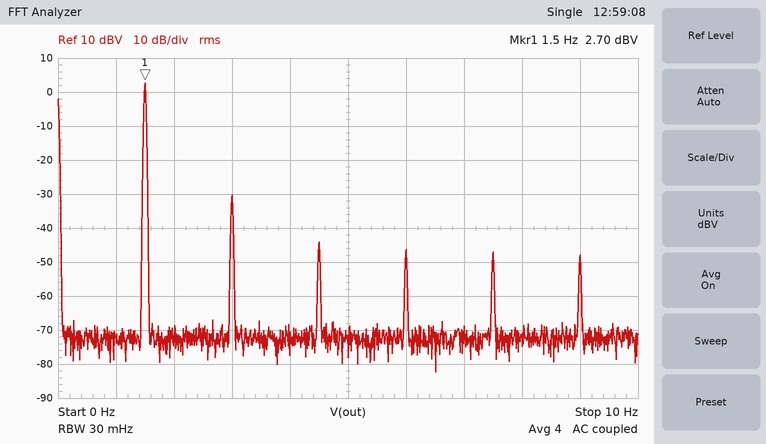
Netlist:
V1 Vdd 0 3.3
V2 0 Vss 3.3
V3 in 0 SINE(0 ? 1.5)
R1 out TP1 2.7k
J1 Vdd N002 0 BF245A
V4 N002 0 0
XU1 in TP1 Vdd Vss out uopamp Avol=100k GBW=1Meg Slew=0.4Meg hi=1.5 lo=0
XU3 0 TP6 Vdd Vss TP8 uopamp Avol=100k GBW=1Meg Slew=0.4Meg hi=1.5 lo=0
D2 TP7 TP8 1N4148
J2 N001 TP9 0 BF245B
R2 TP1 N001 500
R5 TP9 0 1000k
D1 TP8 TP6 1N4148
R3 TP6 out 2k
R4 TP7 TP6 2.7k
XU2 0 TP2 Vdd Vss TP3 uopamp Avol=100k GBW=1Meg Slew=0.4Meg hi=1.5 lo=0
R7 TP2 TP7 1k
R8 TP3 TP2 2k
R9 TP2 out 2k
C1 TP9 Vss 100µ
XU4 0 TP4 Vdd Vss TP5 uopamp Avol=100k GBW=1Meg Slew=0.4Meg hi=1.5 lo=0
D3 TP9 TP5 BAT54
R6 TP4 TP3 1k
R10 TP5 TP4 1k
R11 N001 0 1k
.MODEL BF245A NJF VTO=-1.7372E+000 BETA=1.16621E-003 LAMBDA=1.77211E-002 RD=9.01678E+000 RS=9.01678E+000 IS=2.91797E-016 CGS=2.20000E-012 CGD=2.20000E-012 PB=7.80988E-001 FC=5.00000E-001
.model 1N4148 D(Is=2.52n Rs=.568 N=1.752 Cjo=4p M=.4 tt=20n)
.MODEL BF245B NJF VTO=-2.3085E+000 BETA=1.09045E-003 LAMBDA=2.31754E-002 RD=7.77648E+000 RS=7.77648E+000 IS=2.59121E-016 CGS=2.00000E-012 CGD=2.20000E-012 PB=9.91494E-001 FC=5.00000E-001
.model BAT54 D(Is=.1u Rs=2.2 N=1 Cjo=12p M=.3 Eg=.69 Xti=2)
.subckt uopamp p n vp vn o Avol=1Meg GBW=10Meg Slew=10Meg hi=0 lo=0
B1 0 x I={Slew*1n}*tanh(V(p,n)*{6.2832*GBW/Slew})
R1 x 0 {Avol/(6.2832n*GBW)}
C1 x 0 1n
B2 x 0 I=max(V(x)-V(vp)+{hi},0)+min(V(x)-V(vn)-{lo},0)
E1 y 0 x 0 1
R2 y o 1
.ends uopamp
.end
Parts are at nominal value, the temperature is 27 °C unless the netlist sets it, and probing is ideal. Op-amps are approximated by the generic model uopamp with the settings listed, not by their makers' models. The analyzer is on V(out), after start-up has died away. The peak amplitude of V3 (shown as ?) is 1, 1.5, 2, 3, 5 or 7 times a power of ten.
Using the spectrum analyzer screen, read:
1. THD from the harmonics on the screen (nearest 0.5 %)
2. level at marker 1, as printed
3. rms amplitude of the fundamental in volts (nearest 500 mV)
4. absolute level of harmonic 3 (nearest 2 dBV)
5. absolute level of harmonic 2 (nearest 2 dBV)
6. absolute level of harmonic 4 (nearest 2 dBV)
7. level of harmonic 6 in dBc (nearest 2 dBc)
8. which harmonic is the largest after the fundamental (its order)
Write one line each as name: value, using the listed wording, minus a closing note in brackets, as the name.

THD from the harmonics on the screen: 2.5 %
level at marker 1, as printed: 2.70 dBV
rms amplitude of the fundamental in volts: 1.5 V
absolute level of harmonic 3: -44 dBV
absolute level of harmonic 2: -30 dBV
absolute level of harmonic 4: -46 dBV
level of harmonic 6 in dBc: -50 dBc
which harmonic is the largest after the fundamental: 2
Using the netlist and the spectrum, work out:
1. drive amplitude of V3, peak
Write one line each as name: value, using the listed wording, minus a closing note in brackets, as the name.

drive amplitude of V3, peak: 500 mV
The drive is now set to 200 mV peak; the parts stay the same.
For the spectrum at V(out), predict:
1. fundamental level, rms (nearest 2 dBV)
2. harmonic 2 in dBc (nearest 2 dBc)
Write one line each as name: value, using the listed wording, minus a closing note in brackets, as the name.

fundamental level, rms: -4 dBV
harmonic 2 in dBc: -48 dBc
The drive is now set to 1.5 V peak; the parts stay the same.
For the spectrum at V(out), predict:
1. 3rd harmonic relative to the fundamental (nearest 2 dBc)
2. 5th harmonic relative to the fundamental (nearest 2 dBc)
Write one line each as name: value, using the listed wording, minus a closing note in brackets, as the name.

3rd harmonic relative to the fundamental: -12 dBc
5th harmonic relative to the fundamental: -24 dBc
